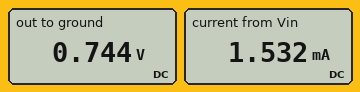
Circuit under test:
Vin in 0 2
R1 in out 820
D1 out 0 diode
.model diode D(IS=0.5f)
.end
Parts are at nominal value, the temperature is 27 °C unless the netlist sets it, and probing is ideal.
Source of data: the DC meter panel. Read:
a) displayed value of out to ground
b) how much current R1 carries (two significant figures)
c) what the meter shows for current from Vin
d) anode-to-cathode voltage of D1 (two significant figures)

0.744 V
1.5 mA
1.532 mA
740 mV
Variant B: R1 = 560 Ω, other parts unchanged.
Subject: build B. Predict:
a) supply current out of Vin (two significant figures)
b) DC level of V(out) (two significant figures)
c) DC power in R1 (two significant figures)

2.2 mA
750 mV
2.8 mW
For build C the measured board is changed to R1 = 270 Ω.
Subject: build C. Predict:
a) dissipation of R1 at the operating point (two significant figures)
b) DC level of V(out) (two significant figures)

5.6 mW
770 mV
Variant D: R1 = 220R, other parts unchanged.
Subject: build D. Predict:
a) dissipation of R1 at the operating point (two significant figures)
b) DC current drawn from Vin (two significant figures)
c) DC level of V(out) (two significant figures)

6.8 mW
5.6 mA
780 mV
